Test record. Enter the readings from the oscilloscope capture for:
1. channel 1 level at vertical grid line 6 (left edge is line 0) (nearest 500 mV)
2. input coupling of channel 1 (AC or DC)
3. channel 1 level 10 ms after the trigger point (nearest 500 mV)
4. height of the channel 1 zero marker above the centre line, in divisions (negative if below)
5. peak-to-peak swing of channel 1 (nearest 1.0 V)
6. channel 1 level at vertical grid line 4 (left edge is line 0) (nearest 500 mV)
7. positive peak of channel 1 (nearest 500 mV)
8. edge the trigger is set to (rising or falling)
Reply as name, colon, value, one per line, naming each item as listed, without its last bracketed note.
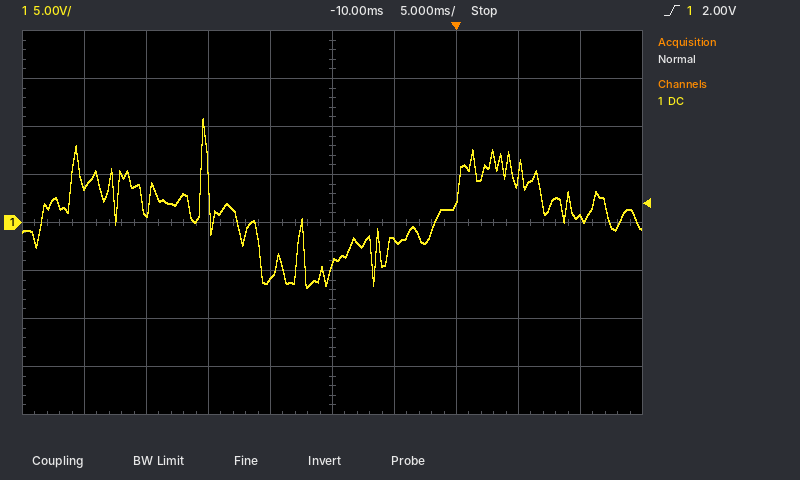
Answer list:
channel 1 level at vertical grid line 6 (left edge is line 0): -2.0 V
input coupling of channel 1: DC
channel 1 level 10 ms after the trigger point: 500 mV
height of the channel 1 zero marker above the centre line, in divisions: 0.0 div
peak-to-peak swing of channel 1: 18.0 V
channel 1 level at vertical grid line 4 (left edge is line 0): -6.0 V
positive peak of channel 1: 11.0 V
edge the trigger is set to: rising
